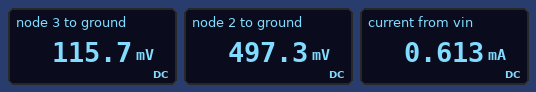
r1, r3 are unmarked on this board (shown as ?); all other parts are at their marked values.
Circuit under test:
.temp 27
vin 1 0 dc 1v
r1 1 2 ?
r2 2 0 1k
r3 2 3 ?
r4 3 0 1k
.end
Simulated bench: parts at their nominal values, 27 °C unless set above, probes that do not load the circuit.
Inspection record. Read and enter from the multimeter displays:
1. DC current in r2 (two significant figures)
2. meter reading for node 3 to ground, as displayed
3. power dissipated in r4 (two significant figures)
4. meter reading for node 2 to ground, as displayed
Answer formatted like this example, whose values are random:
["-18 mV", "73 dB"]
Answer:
["500 µA", "115.7 mV", "13 µW", "497.3 mV"]
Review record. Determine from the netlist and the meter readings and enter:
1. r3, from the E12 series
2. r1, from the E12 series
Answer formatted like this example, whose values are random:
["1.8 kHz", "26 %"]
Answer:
["3.3 kΩ", "820 Ω"]
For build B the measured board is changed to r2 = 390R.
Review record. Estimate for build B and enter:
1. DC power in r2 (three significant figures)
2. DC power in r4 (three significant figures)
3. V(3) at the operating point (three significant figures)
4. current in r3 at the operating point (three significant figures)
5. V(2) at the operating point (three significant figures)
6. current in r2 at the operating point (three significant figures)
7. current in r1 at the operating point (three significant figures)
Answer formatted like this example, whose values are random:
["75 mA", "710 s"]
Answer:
["236 µW", "4.99 µW", "70.6 mV", "70.6 µA", "304 mV", "779 µA", "849 µA"]
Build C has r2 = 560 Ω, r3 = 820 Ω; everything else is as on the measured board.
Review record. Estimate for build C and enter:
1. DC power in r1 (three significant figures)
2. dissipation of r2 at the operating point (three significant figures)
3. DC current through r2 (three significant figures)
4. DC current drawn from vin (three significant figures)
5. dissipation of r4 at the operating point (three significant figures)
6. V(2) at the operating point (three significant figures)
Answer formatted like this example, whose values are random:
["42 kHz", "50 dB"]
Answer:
["526 µW", "210 µW", "613 µA", "801 µA", "35.5 µW", "343 mV"]
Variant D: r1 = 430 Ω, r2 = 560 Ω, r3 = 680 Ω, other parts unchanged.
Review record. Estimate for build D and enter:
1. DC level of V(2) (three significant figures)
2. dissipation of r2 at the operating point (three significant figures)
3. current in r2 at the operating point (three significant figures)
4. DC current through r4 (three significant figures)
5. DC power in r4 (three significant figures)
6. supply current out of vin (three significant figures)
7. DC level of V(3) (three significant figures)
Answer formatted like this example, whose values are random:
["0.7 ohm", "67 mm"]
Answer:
["494 mV", "436 µW", "882 µA", "294 µA", "86.5 µW", "1.18 mA", "294 mV"]
